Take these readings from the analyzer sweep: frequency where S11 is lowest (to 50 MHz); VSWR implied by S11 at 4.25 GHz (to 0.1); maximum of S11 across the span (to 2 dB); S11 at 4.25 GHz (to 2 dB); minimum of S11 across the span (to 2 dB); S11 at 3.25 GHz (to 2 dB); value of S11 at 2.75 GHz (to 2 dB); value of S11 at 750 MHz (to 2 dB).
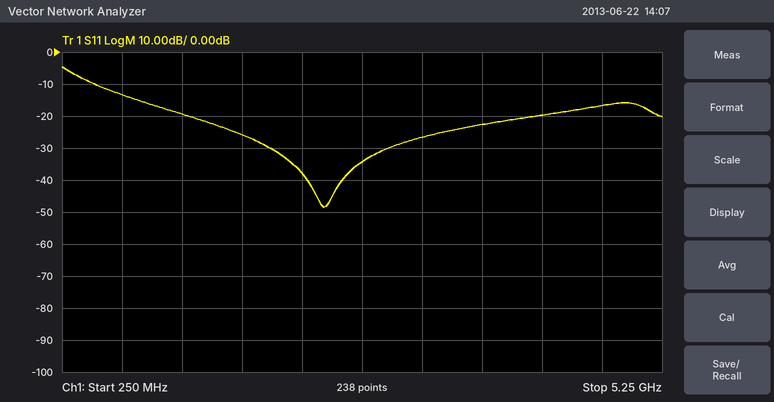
2.45 GHz
1.2
-4 dB
-20 dB
-48 dB
-26 dB
-34 dB
-14 dB
